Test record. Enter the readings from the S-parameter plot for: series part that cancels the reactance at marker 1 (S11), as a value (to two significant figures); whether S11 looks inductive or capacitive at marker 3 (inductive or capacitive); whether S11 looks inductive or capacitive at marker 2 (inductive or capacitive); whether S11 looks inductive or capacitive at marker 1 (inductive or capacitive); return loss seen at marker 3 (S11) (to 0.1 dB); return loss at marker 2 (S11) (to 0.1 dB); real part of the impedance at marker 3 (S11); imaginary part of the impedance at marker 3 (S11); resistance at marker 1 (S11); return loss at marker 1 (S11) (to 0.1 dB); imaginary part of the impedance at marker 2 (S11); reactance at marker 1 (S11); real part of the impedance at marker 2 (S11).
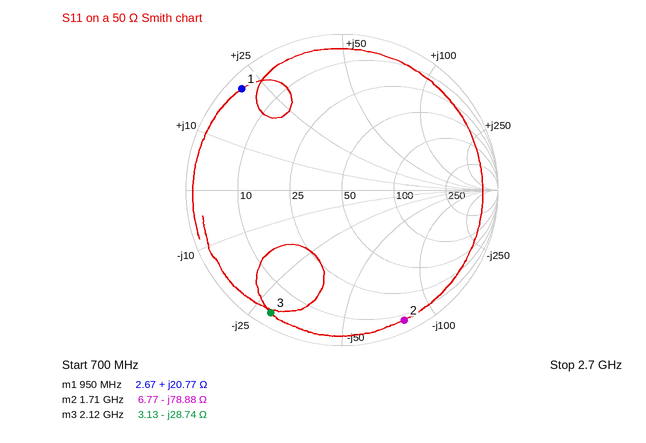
8.1 pF
capacitive
capacitive
inductive
0.8 dB
0.7 dB
3.13 Ω
-28.74 Ω
2.67 Ω
0.8 dB
-78.88 Ω
+20.77 Ω
6.77 Ω
